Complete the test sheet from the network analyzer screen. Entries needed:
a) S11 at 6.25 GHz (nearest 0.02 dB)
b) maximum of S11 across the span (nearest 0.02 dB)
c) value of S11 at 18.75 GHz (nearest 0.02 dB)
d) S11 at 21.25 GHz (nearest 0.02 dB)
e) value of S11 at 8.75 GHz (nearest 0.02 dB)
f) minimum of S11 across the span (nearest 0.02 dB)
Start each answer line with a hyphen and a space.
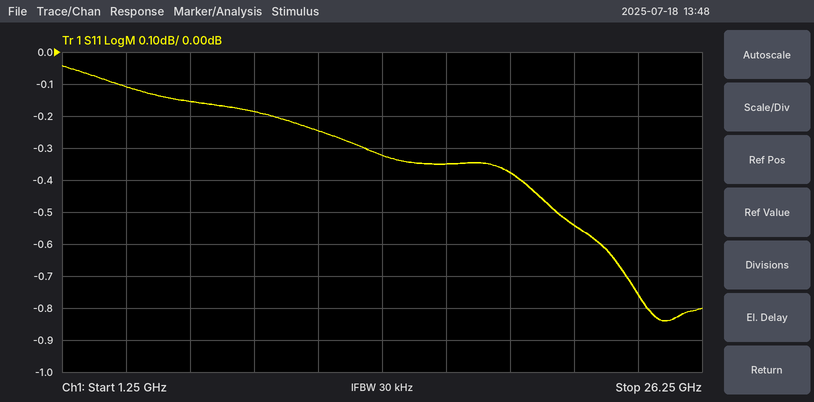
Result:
- -0.16 dB
- -0.04 dB
- -0.38 dB
- -0.54 dB
- -0.18 dB
- -0.84 dB
